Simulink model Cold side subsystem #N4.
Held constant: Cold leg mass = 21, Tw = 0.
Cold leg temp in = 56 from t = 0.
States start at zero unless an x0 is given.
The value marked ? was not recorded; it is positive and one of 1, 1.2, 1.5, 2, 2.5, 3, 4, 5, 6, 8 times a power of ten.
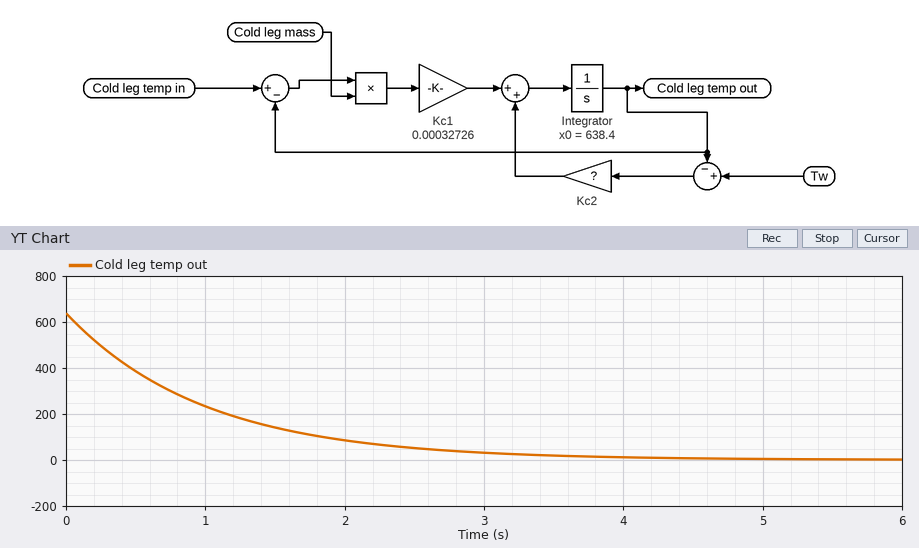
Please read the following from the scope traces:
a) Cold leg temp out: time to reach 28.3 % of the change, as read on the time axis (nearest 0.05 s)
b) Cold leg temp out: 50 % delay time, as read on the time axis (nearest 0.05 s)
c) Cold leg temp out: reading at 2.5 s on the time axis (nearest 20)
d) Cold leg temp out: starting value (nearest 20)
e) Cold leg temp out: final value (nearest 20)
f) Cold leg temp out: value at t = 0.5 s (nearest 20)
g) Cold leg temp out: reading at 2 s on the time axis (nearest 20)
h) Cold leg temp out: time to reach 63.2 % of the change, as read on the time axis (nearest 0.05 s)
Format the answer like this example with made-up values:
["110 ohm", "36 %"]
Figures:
["0.35 s", "0.70 s", "60", "640", "0", "380", "80", "1.00 s"]
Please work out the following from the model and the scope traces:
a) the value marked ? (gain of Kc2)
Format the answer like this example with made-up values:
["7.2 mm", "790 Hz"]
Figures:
["1"]
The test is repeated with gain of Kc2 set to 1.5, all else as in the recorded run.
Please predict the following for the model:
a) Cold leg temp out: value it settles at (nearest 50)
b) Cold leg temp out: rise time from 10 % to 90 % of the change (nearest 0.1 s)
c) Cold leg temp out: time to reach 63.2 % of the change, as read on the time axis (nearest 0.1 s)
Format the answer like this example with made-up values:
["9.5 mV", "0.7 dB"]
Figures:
["0", "1.5 s", "0.7 s"]
